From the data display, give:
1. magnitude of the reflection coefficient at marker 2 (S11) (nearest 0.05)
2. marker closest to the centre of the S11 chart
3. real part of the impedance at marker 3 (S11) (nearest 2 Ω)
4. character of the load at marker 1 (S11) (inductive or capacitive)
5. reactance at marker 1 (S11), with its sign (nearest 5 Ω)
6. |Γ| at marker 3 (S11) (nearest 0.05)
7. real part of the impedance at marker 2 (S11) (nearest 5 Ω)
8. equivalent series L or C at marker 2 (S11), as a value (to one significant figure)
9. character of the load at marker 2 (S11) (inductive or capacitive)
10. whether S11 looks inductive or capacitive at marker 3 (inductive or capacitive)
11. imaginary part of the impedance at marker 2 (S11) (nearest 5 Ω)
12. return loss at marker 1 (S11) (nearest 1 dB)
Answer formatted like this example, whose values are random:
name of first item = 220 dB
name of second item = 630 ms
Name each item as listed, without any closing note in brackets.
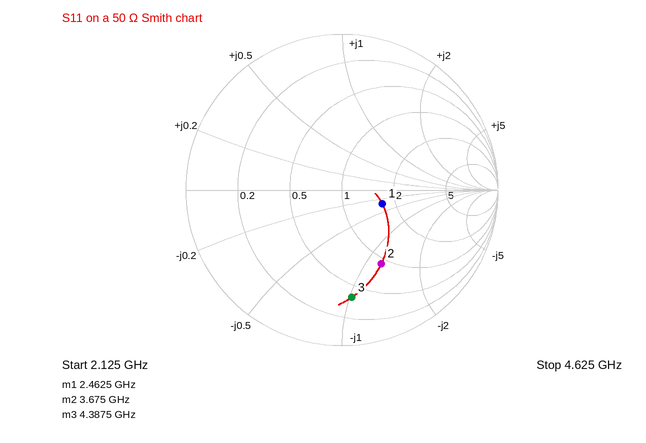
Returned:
magnitude of the reflection coefficient at marker 2 (S11) = 0.55
marker closest to the centre of the S11 chart = marker 1
real part of the impedance at marker 3 (S11) = 20 Ω
character of the load at marker 1 (S11) = capacitive
reactance at marker 1 (S11), with its sign = -15 Ω
|Γ| at marker 3 (S11) = 0.70
real part of the impedance at marker 2 (S11) = 45 Ω
equivalent series L or C at marker 2 (S11), as a value = 700 fF
character of the load at marker 2 (S11) = capacitive
whether S11 looks inductive or capacitive at marker 3 = capacitive
imaginary part of the impedance at marker 2 (S11) = -60 Ω
return loss at marker 1 (S11) = 11 dB
